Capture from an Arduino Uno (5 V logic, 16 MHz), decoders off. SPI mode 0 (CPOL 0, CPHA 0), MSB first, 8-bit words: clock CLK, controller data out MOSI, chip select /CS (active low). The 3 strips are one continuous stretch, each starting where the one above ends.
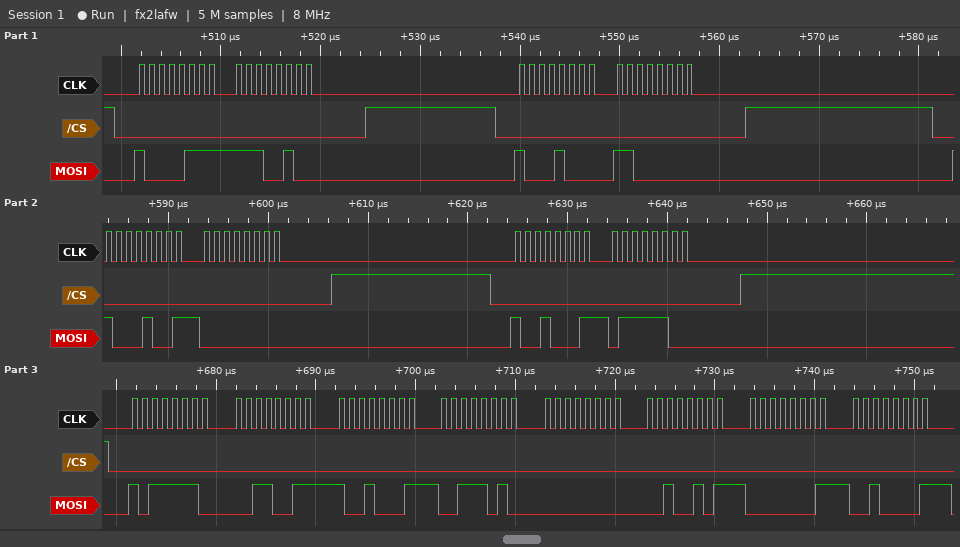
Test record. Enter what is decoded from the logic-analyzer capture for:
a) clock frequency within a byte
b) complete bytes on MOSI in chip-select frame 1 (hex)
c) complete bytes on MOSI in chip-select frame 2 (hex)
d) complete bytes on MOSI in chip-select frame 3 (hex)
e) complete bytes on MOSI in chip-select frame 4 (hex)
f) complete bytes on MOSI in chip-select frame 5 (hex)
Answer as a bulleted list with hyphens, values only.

- 1 MHz
- 87 E4
- 88 C0
- 89 00
- 91 7C
- BE 33 91 3A 00 25 01 21
